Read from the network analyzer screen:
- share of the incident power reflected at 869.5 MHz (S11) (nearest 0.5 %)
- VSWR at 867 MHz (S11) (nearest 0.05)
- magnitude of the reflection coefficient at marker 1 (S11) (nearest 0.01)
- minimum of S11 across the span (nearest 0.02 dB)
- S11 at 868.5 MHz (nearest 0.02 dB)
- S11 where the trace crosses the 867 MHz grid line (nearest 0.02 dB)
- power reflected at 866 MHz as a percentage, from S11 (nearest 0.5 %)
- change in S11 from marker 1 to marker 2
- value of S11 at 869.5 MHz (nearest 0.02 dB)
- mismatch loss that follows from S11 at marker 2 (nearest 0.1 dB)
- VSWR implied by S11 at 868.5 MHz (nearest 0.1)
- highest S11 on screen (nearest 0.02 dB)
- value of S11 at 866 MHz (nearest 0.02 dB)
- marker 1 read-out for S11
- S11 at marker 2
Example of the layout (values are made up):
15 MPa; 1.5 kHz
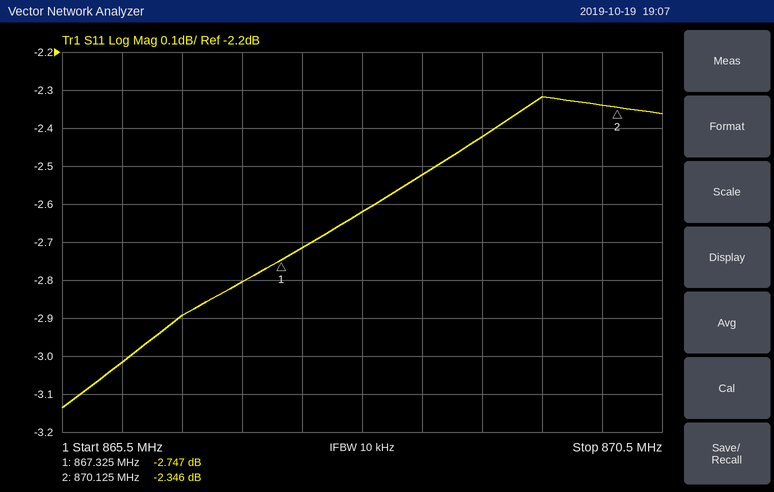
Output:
58.5 %; 6.25; 0.73; -3.14 dB; -2.52 dB; -2.80 dB; 50.0 %; 0.401 dB; -2.32 dB; 3.8 dB; 6.9; -2.32 dB; -3.02 dB; -2.747 dB; -2.346 dB
